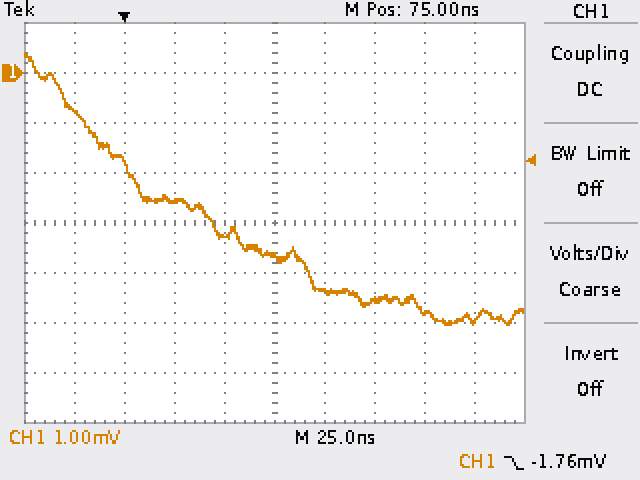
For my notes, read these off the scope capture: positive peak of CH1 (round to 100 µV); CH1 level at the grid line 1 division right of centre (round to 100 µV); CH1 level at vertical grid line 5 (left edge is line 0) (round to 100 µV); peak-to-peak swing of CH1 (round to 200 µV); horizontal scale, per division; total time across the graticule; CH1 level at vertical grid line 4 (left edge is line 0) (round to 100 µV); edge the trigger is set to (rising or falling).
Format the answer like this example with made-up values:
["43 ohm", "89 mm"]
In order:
["400 µV", "-4.4 mV", "-3.7 mV", "5.4 mV", "25 ns", "250 ns", "-3.3 mV", "falling"]
